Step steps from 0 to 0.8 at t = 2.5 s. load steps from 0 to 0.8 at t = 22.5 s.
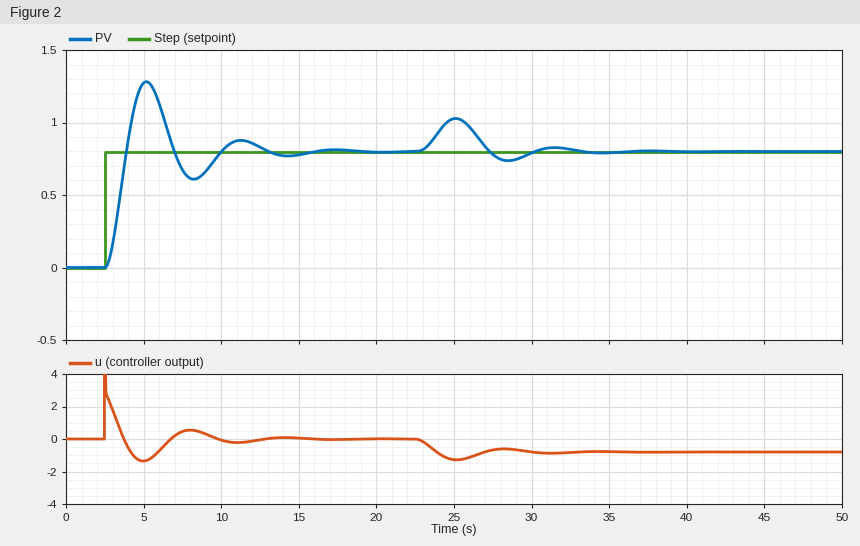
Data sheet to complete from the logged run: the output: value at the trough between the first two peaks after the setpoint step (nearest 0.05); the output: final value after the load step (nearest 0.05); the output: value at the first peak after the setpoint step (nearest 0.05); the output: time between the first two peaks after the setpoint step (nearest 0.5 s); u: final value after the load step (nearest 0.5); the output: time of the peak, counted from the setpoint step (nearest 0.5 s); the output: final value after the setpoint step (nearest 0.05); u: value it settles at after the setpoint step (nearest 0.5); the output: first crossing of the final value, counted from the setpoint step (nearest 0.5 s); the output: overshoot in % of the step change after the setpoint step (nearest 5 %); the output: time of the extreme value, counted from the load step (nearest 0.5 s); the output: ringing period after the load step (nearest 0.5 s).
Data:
0.60
0.80
1.30
6.0 s
-1.0
2.5 s
0.80
0.0
1.5 s
60 %
2.5 s
6.5 s
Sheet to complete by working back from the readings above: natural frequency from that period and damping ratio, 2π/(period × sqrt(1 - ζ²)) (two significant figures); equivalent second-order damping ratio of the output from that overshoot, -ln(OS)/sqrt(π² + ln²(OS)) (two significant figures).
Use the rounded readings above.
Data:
1.1 rad/s
0.16
